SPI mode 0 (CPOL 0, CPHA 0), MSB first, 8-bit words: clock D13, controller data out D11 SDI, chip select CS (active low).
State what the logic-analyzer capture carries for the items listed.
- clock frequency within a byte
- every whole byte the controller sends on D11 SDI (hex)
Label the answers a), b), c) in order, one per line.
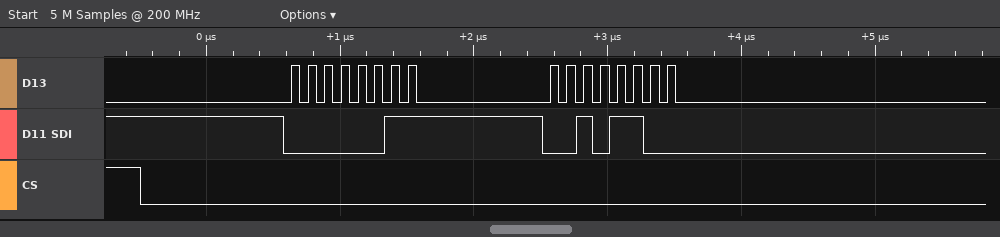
a) 8 MHz
b) 03 2C
